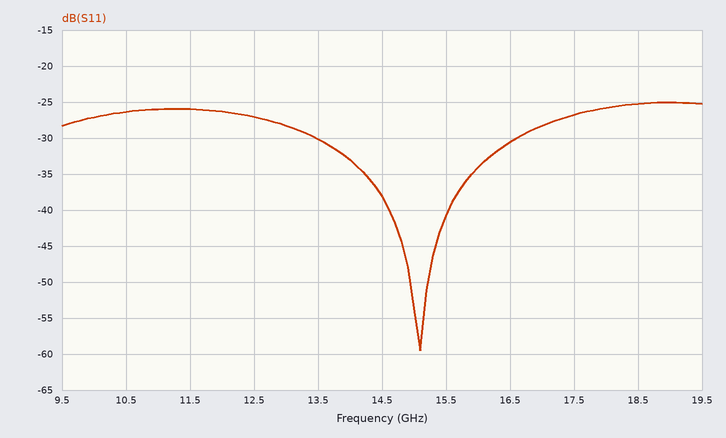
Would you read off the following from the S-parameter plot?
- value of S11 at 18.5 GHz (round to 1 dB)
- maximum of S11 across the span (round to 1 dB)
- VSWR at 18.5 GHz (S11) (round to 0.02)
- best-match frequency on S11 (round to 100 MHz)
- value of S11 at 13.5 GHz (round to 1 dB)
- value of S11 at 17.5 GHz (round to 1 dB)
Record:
-25 dB
-25 dB
1.12
15.1 GHz
-30 dB
-27 dB
